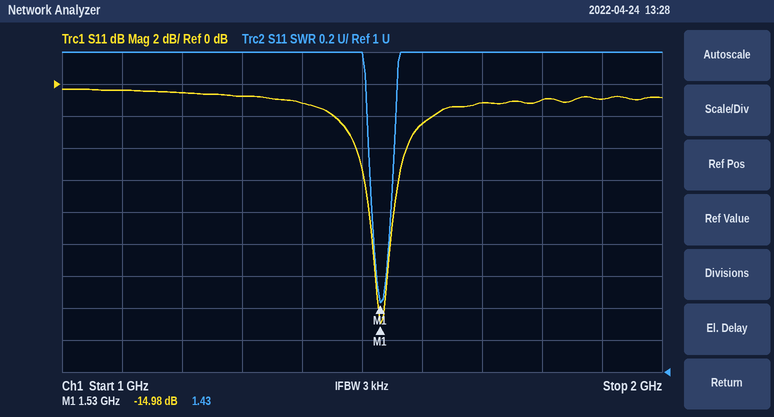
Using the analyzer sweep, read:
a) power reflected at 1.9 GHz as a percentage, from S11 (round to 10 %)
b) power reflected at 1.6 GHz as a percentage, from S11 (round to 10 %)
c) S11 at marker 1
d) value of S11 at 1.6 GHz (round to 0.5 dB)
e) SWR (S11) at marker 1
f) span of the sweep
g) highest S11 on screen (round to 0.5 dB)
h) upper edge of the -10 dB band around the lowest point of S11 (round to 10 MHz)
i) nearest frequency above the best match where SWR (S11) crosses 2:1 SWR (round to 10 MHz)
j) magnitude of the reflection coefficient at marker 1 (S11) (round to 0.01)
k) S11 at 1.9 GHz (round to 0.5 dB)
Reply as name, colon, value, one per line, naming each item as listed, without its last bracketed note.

power reflected at 1.9 GHz as a percentage, from S11: 80 %
power reflected at 1.6 GHz as a percentage, from S11: 60 %
S11 at marker 1: -14.98 dB
value of S11 at 1.6 GHz: -2.5 dB
SWR (S11) at marker 1: 1.43
span of the sweep: 1 GHz
highest S11 on screen: -0.5 dB
upper edge of the -10 dB band around the lowest point of S11: 1.55 GHz
nearest frequency above the best match where SWR (S11) crosses 2:1 SWR: 1.55 GHz
magnitude of the reflection coefficient at marker 1 (S11): 0.18
S11 at 1.9 GHz: -1.0 dB
